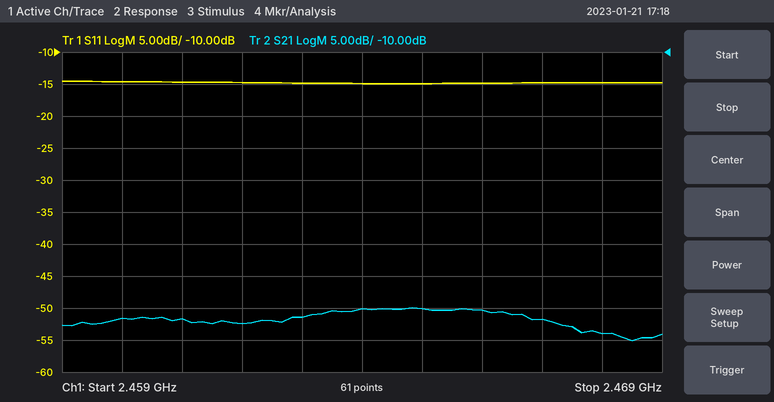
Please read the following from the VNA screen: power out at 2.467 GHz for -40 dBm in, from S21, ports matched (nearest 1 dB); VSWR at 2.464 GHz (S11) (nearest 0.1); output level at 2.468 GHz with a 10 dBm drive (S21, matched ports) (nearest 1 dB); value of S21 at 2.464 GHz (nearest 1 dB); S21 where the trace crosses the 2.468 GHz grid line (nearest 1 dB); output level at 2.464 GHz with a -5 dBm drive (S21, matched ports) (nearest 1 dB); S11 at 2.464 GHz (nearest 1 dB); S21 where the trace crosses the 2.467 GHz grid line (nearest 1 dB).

-92 dBm
1.4
-44 dBm
-50 dB
-54 dB
-55 dBm
-15 dB
-52 dB
